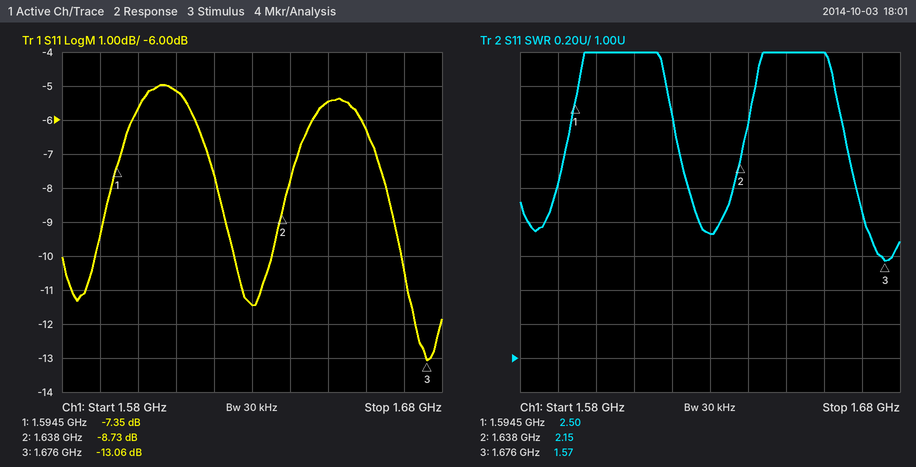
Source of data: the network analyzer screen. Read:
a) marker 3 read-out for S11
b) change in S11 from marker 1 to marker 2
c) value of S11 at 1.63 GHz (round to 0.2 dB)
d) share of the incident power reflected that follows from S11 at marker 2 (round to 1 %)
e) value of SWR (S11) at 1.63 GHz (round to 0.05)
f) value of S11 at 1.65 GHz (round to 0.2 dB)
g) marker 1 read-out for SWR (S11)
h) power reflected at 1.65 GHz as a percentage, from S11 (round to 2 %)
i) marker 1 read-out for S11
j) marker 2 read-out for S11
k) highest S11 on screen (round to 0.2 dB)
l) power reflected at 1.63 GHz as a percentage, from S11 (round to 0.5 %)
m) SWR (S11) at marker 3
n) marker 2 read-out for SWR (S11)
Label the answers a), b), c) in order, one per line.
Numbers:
a) -13.06 dB
b) -1.38 dB
c) -11.4 dB
d) 13 %
e) 1.75
f) -5.4 dB
g) 2.50
h) 28 %
i) -7.35 dB
j) -8.73 dB
k) -5.0 dB
l) 7.0 %
m) 1.57
n) 2.15
